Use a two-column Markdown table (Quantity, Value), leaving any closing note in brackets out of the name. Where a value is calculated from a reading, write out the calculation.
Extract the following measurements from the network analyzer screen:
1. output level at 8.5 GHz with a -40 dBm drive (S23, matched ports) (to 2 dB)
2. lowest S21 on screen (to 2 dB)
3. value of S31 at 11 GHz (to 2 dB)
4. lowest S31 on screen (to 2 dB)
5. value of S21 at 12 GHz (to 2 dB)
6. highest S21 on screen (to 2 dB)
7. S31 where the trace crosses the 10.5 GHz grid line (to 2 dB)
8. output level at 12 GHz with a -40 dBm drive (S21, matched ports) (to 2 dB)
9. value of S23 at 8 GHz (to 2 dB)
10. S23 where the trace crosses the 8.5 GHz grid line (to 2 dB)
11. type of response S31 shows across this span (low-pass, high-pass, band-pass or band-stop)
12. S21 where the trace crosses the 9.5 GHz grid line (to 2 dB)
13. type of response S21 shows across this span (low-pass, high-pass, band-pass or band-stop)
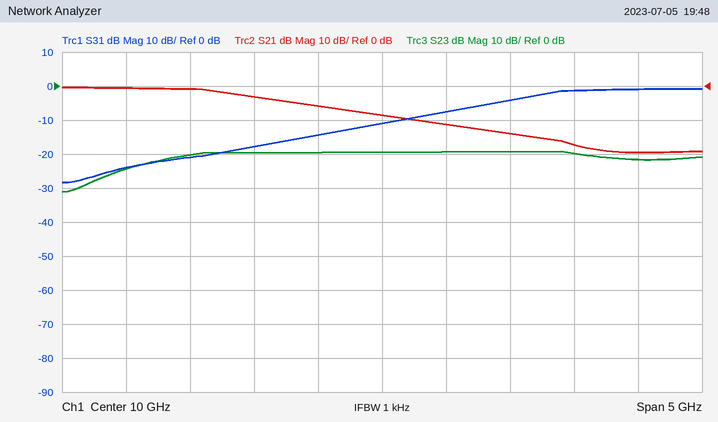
| Quantity | Value |
|---|---|
| output level at 8.5 GHz with a -40 dBm drive (S23, matched ports) | -40 dBm + (-20 dB) = -60 dBm |
| lowest S21 on screen | -20 dB |
| value of S31 at 11 GHz | -4 dB |
| lowest S31 on screen | -28 dB |
| value of S21 at 12 GHz | -20 dB |
| highest S21 on screen | 0 dB |
| S31 where the trace crosses the 10.5 GHz grid line | -8 dB |
| output level at 12 GHz with a -40 dBm drive (S21, matched ports) | -40 dBm + (-20 dB) = -60 dBm |
| value of S23 at 8 GHz | -24 dB |
| S23 where the trace crosses the 8.5 GHz grid line | -20 dB |
| type of response S31 shows across this span | high-pass |
| S21 where the trace crosses the 9.5 GHz grid line | -6 dB |
| type of response S21 shows across this span | low-pass |
